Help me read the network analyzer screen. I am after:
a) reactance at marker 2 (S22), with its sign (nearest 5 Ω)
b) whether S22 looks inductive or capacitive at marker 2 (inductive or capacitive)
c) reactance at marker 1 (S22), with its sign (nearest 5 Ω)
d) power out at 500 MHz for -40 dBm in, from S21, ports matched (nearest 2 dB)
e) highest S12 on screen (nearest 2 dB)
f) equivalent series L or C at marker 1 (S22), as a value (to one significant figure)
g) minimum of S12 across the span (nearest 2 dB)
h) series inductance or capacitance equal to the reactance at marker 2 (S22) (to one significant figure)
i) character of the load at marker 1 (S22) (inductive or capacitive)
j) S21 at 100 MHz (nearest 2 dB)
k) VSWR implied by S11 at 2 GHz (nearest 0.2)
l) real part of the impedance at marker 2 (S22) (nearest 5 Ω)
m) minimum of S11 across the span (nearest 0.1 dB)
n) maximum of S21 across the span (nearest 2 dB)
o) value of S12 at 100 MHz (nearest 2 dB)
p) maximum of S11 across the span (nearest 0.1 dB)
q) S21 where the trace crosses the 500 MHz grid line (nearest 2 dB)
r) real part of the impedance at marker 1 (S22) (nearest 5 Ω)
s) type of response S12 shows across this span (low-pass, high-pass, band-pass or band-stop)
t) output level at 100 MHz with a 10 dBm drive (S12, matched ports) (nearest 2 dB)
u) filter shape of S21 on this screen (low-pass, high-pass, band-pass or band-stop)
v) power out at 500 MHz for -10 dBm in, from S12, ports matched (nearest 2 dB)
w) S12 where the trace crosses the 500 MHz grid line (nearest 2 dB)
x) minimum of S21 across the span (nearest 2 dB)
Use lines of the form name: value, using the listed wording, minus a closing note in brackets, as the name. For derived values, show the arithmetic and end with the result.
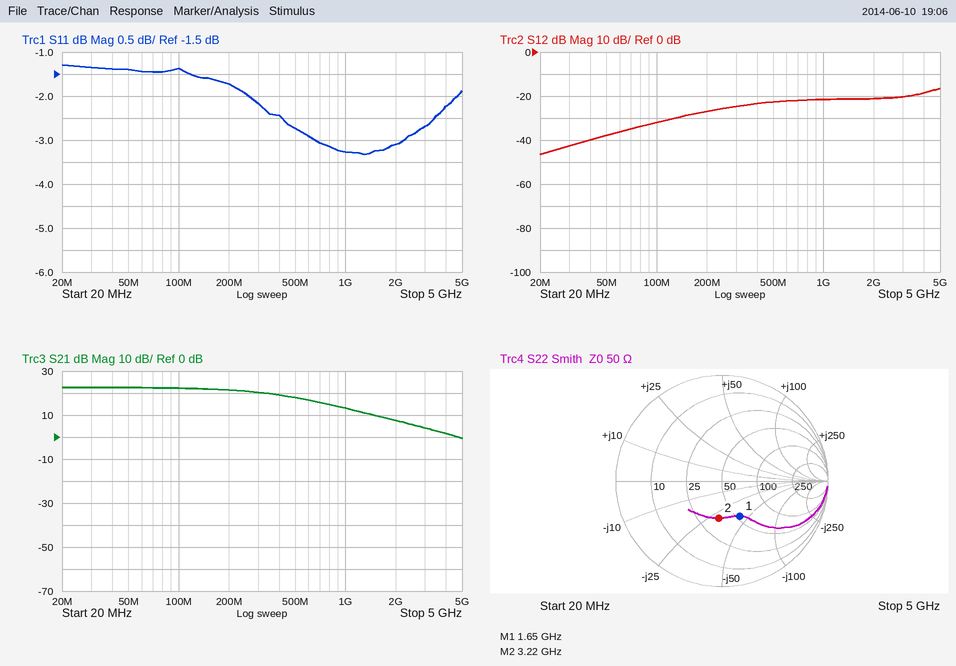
reactance at marker 2 (S22), with its sign: -30 Ω
whether S22 looks inductive or capacitive at marker 2: capacitive
reactance at marker 1 (S22), with its sign: -40 Ω
power out at 500 MHz for -40 dBm in, from S21, ports matched: -40 dBm + (18 dB) = -22 dBm
highest S12 on screen: -16 dB
equivalent series L or C at marker 1 (S22), as a value: C = 1/(2π × 1.65 GHz × 40 Ω) ≈ 2 pF
minimum of S12 across the span: -46 dB
series inductance or capacitance equal to the reactance at marker 2 (S22): C = 1/(2π × 3.22 GHz × 30 Ω) ≈ 2 pF
character of the load at marker 1 (S22): capacitive
S21 at 100 MHz: 22 dB
VSWR implied by S11 at 2 GHz: |Γ| = 10^(-3.1/20) = 0.6998; VSWR = (1 + 0.6998)/(1 − 0.6998) ≈ 5.66, so 5.6 to the nearest 0.2
real part of the impedance at marker 2 (S22): 35 Ω
minimum of S11 across the span: -3.3 dB
maximum of S21 across the span: 22 dB
value of S12 at 100 MHz: -32 dB
maximum of S11 across the span: -1.3 dB
S21 where the trace crosses the 500 MHz grid line: 18 dB
real part of the impedance at marker 1 (S22): 55 Ω
type of response S12 shows across this span: high-pass
output level at 100 MHz with a 10 dBm drive (S12, matched ports): 10 dBm + (-32 dB) = -22 dBm
filter shape of S21 on this screen: low-pass
power out at 500 MHz for -10 dBm in, from S12, ports matched: -10 dBm + (-22 dB) = -32 dBm
S12 where the trace crosses the 500 MHz grid line: -22 dB
minimum of S21 across the span: 0 dB
